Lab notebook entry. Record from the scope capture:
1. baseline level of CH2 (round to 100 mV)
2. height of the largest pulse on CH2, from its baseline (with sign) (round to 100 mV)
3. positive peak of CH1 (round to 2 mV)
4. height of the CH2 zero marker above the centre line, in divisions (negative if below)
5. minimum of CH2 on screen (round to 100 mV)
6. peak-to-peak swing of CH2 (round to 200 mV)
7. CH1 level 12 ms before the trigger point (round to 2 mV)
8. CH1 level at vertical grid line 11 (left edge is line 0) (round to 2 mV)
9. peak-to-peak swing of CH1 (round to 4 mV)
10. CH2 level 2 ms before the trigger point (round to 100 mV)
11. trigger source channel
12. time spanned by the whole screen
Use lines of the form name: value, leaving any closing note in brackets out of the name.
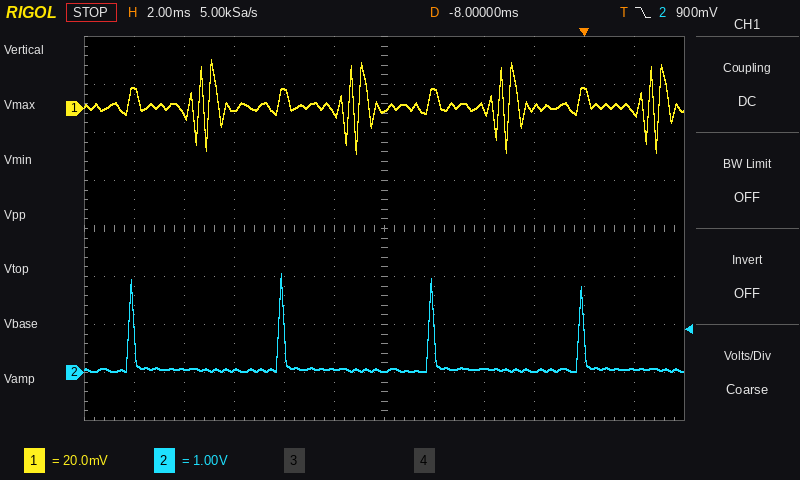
baseline level of CH2: 100 mV
height of the largest pulse on CH2, from its baseline (with sign): +2.0 V
positive peak of CH1: 20 mV
height of the CH2 zero marker above the centre line, in divisions: -3.0 div
minimum of CH2 on screen: 0.0 V
peak-to-peak swing of CH2: 2.0 V
CH1 level 12 ms before the trigger point: 8 mV
CH1 level at vertical grid line 11 (left edge is line 0): -2 mV
peak-to-peak swing of CH1: 40 mV
CH2 level 2 ms before the trigger point: 0.0 V
trigger source channel: CH2
time spanned by the whole screen: 24 ms
